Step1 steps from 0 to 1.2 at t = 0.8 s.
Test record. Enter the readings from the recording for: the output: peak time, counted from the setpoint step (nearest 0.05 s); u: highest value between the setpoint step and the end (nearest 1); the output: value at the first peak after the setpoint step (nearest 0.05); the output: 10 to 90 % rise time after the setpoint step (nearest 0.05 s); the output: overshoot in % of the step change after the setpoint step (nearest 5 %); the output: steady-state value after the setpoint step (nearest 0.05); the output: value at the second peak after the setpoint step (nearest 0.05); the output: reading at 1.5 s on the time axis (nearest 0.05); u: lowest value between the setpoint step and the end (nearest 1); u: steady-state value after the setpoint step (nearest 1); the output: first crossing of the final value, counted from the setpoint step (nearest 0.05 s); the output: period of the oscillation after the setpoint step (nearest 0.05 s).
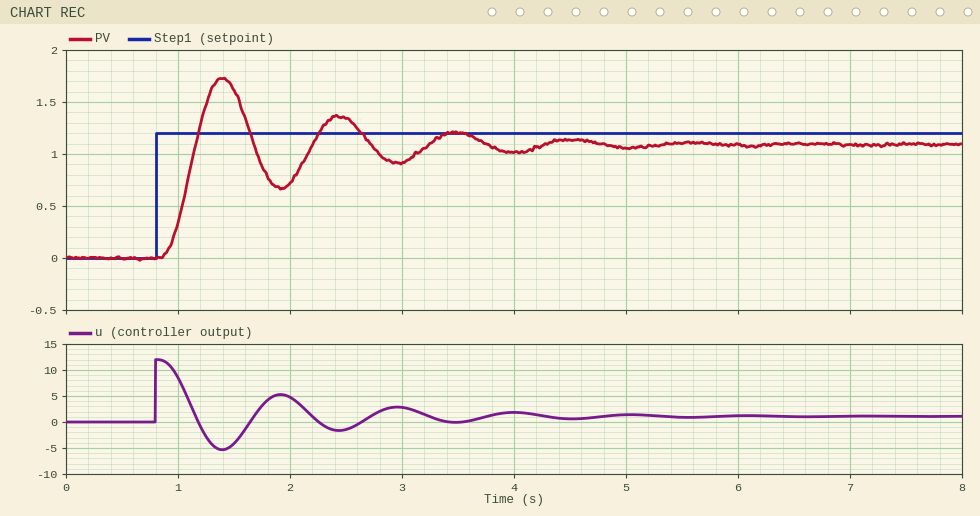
0.60 s
12
1.75
0.20 s
60 %
1.10
1.35
1.60
-5
1
0.35 s
1.05 s
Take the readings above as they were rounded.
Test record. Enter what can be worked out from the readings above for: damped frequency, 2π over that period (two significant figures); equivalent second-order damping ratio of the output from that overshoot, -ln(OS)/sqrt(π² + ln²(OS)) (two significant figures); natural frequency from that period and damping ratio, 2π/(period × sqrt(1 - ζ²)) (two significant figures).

6.0 rad/s
0.16
6.1 rad/s
